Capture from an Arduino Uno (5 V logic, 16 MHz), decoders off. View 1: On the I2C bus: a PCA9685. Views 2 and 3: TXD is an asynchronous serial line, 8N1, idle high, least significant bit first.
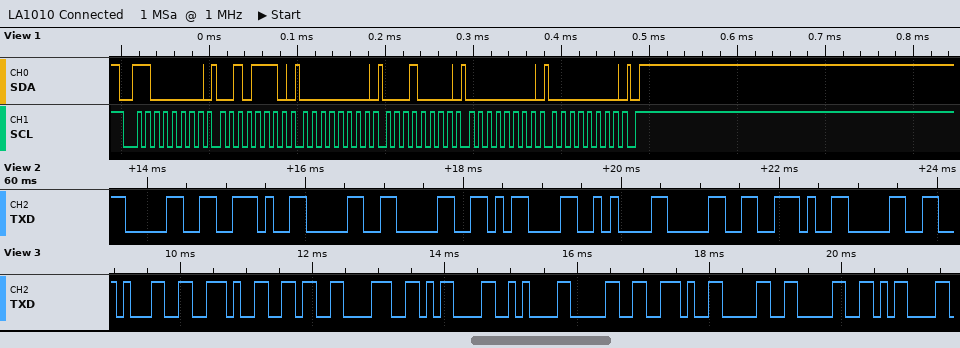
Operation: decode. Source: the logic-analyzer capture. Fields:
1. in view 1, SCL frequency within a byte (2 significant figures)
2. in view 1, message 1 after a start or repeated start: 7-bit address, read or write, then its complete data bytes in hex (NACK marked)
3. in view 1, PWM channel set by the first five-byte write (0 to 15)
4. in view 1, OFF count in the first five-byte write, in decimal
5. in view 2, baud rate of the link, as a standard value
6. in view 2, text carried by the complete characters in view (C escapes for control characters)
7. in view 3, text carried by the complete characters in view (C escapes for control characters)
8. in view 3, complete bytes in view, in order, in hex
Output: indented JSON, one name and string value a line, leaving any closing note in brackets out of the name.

{
  "in view 1, SCL frequency within a byte": "100 kHz",
  "in view 1, message 1 after a start or repeated start: 7-bit address, read or write, then its complete data bytes in hex": "0x60 write: 2E 00 10 00 00",
  "in view 1, PWM channel set by the first five-byte write": "10",
  "in view 1, OFF count in the first five-byte write, in decimal": "0",
  "in view 2, baud rate of the link, as a standard value": "9600 baud",
  "in view 2, text carried by the complete characters in view": "\"0.00\\r\\n0.0\"",
  "in view 3, text carried by the complete characters in view": "\"1.68\\r\\n0.00\\r\"",
  "in view 3, complete bytes in view, in order, in hex": "31 2E 36 38 0D 0A 30 2E 30 30 0D"
}
